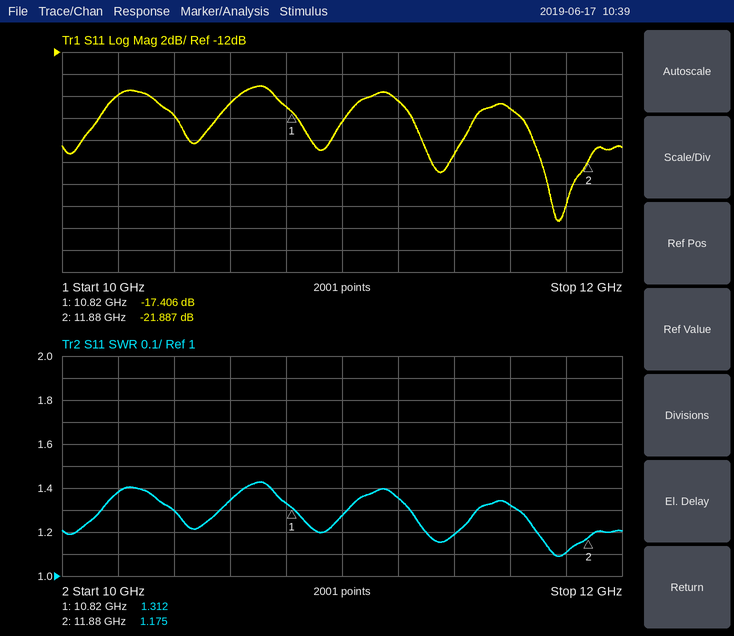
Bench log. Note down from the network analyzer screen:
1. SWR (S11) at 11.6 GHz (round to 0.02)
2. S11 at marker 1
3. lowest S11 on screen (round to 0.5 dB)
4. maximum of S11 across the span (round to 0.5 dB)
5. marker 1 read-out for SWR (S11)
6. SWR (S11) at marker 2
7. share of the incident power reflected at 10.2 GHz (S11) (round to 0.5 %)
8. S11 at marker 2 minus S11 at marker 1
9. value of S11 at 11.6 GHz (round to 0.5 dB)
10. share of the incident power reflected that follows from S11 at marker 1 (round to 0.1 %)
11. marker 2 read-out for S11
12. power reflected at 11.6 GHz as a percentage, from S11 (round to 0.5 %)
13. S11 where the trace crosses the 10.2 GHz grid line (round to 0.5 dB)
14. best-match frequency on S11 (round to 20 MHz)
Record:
1.32
-17.406 dB
-27.5 dB
-15.0 dB
1.312
1.175
2.5 %
-4.481 dB
-17.0 dB
1.8 %
-21.887 dB
2.0 %
-16.0 dB
11.78 GHz
